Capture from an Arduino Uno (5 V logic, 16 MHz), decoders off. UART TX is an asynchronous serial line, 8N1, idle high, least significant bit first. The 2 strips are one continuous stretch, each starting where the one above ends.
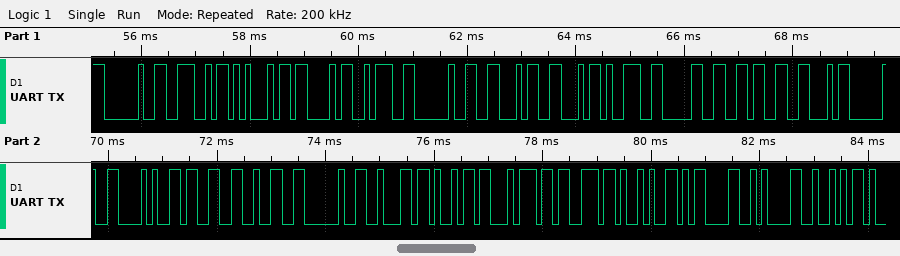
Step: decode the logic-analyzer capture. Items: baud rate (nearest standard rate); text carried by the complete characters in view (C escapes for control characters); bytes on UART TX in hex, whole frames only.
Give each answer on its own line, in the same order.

9600 baud
" NEC: FF906F (32 bits)\r\nR"
20 4E 45 43 3A 20 46 46 39 30 36 46 20 28 33 32 20 62 69 74 73 29 0D 0A 52
